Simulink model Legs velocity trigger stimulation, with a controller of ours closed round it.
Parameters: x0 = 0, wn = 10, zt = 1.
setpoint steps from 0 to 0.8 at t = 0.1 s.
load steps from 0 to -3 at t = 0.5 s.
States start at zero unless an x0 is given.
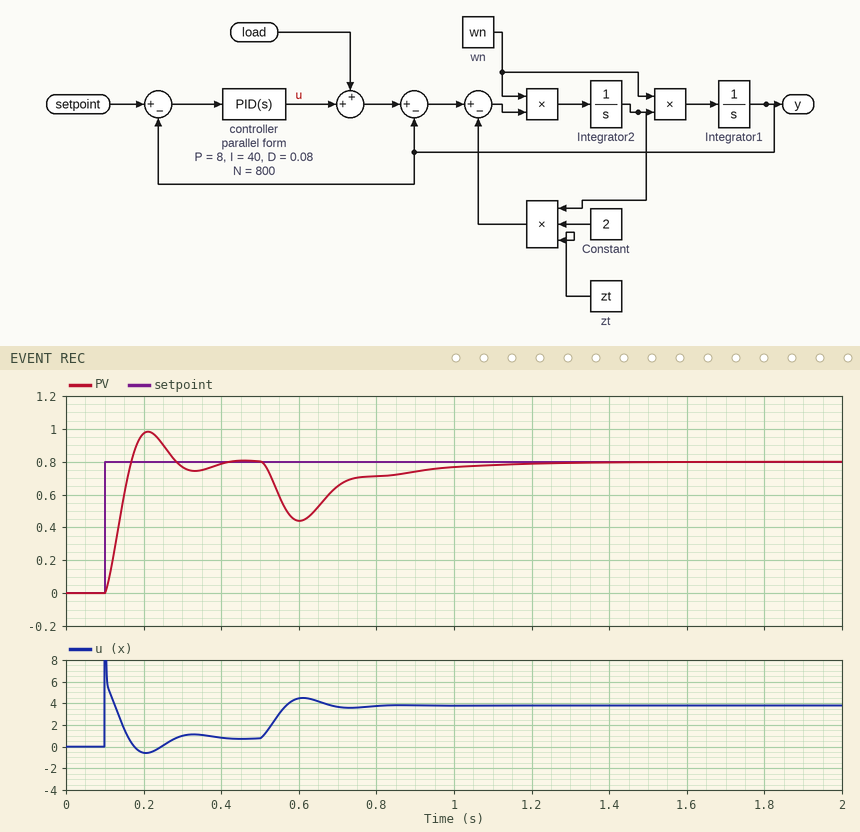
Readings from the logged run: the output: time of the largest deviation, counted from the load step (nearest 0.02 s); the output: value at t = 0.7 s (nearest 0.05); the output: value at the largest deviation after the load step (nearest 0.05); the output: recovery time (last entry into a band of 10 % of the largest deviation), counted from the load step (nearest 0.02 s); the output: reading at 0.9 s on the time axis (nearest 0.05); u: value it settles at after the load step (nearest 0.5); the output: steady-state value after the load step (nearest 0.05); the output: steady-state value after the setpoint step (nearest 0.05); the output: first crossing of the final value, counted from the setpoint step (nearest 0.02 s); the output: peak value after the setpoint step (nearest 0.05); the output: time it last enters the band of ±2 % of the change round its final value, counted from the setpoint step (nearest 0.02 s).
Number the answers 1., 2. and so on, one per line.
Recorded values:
1. 0.10 s
2. 0.65
3. 0.45
4. 0.48 s
5. 0.75
6. 4.0
7. 0.80
8. 0.80
9. 0.06 s
10. 1.00
11. 0.30 s
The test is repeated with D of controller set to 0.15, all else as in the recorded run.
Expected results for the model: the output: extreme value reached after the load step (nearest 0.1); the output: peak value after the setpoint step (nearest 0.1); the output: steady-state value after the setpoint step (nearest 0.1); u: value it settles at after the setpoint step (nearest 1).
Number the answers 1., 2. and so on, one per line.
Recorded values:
1. 0.5
2. 0.9
3. 0.8
4. 1
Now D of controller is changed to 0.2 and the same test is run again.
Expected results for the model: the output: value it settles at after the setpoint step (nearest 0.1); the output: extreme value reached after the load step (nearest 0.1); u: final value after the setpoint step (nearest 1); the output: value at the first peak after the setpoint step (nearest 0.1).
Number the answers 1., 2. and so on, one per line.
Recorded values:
1. 0.8
2. 0.5
3. 1
4. 0.9
